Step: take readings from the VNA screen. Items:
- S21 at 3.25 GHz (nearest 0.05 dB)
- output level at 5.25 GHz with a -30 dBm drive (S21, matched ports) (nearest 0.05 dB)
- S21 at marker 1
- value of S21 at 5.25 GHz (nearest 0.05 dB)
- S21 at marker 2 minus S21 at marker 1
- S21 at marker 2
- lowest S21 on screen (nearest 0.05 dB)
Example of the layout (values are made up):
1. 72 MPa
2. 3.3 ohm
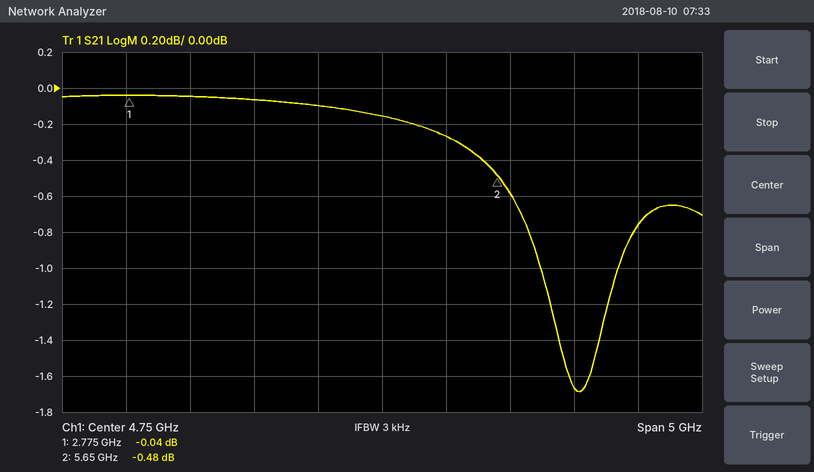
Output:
1. -0.05 dB
2. -30.25 dBm
3. -0.04 dB
4. -0.25 dB
5. -0.44 dB
6. -0.48 dB
7. -1.70 dB
